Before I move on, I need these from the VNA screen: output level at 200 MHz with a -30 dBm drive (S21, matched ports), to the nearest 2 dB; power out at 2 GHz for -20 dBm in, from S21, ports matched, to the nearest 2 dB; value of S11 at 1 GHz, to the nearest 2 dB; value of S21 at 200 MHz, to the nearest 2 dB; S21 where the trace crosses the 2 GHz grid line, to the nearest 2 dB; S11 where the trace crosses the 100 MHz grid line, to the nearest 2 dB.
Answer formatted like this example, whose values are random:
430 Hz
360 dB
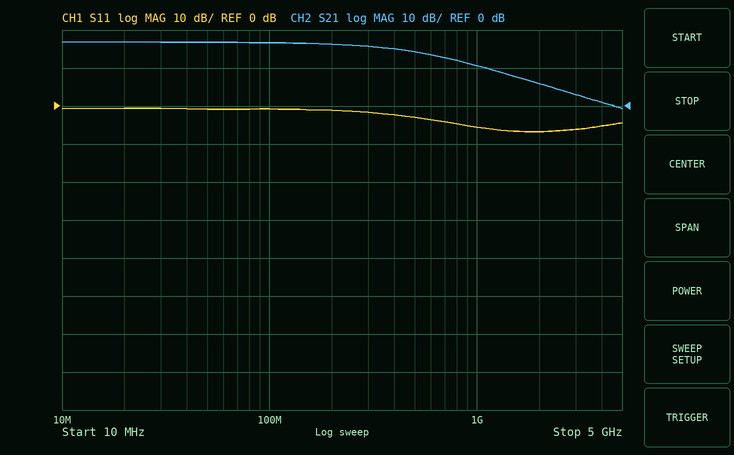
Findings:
-14 dBm
-14 dBm
-6 dB
16 dB
6 dB
0 dB
